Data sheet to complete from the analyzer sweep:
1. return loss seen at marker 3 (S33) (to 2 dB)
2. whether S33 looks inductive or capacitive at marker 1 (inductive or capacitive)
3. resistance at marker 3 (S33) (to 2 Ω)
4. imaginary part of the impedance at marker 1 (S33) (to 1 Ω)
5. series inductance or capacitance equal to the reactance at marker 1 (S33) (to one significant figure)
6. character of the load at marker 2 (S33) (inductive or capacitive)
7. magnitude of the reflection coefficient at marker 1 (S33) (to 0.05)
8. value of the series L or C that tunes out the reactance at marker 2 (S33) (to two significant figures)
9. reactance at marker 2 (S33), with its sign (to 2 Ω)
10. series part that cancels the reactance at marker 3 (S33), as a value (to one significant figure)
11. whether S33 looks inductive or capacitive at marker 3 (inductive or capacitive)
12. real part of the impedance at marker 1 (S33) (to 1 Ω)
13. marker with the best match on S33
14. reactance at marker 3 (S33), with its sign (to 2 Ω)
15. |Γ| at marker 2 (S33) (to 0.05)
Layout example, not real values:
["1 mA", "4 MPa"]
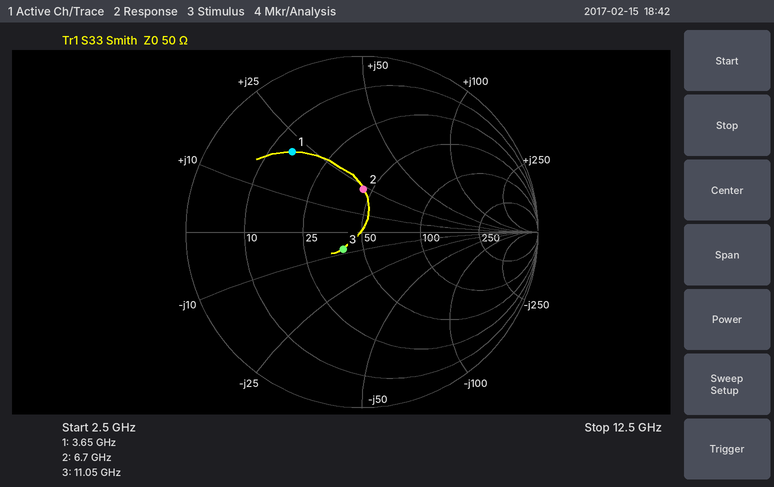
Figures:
["16 dB", "inductive", "40 Ω", "+21 Ω", "900 pH", "inductive", "0.60", "1.0 pF", "+24 Ω", "100 pH", "capacitive", "15 Ω", "marker 3", "-8 Ω", "0.25"]
